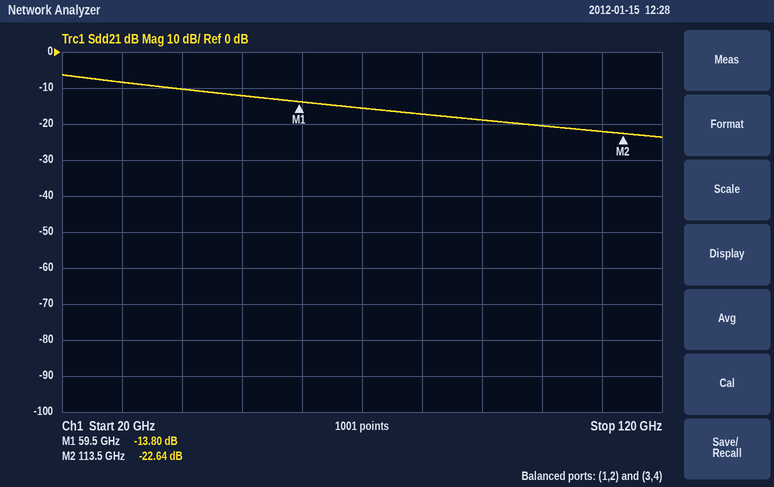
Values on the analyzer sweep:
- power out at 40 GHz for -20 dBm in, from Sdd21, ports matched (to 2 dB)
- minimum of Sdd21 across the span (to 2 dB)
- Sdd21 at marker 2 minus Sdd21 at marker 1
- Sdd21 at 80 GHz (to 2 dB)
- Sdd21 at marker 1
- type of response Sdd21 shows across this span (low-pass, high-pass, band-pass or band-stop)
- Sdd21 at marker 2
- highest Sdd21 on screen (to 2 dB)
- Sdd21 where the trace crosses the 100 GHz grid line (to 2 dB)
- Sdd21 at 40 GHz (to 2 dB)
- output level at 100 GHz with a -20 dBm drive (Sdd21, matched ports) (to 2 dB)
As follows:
-30 dBm
-24 dB
-8.84 dB
-18 dB
-13.80 dB
low-pass
-22.64 dB
-6 dB
-20 dB
-10 dB
-40 dBm
